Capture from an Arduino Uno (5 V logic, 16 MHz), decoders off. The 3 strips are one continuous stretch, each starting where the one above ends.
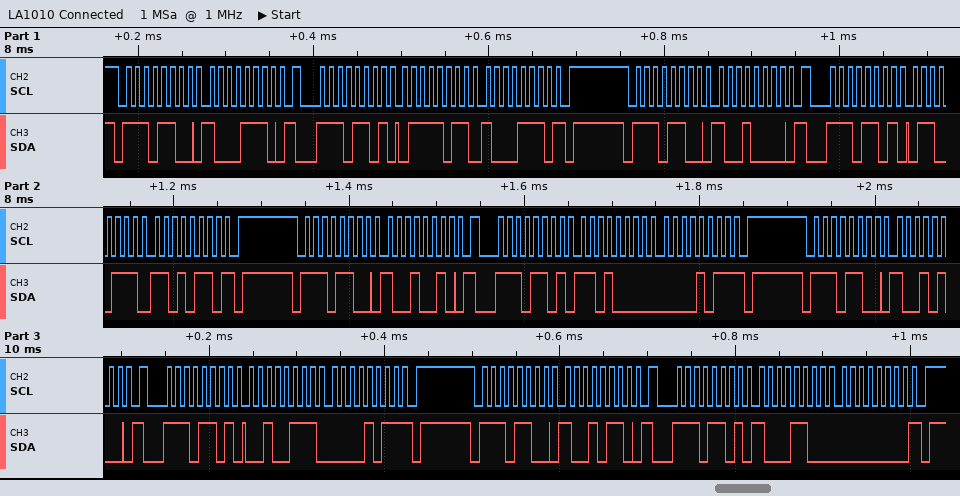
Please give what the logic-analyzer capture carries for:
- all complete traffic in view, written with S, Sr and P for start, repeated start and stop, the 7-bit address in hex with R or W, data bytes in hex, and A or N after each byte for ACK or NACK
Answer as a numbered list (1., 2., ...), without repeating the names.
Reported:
1. S 76W A 8E A Sr 76R A 7B A 8E N P S 76W A 90 A Sr 76R A 67 A D6 N P S 76W A 92 A Sr 76R A D0 A 0B N P S 76W A 94 A Sr 76R A 27 A 0B N P S 76W A 96 A Sr 76R A 8C A 00 N P
